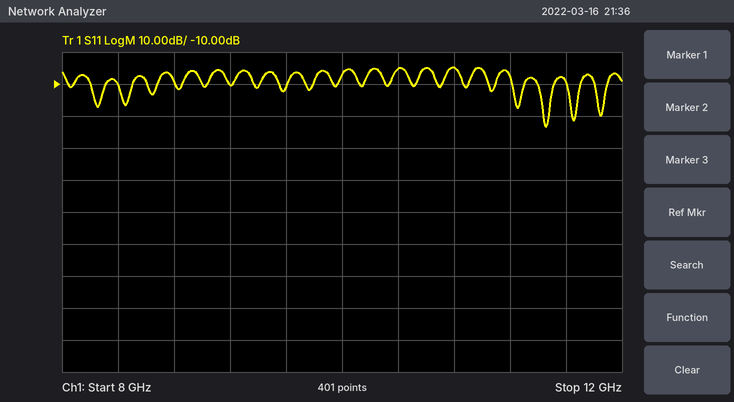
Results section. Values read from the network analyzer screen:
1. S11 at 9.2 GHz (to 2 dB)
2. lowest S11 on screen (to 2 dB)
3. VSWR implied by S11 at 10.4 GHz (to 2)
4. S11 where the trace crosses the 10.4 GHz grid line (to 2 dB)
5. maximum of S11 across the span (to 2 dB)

-10 dB
-24 dB
4
-6 dB
-4 dB
